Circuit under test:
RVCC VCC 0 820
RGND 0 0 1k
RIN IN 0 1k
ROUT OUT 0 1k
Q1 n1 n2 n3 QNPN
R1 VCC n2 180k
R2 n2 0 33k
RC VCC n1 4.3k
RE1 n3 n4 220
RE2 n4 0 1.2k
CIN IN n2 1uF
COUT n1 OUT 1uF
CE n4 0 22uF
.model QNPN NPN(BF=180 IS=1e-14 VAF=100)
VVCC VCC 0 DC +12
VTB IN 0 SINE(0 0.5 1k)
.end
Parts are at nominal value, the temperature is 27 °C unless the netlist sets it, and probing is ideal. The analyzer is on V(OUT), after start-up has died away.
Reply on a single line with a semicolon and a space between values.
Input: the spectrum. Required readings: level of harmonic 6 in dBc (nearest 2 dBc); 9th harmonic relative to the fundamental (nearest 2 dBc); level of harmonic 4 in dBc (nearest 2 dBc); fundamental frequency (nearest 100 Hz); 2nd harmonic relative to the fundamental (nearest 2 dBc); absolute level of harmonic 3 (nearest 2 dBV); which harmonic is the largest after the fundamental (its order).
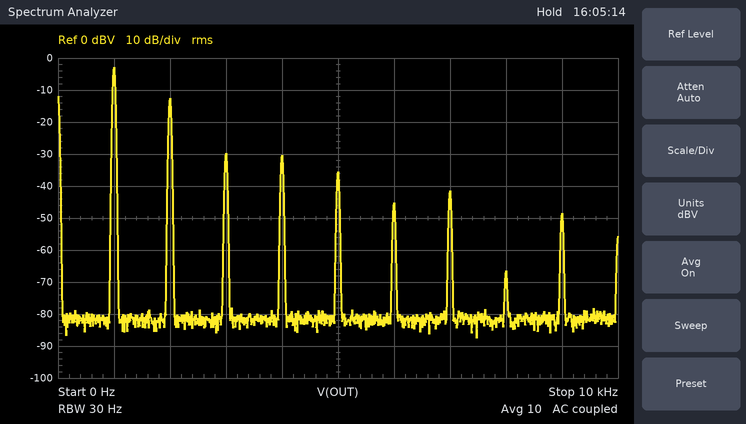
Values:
-42 dBc; -46 dBc; -28 dBc; 1.0 kHz; -10 dBc; -30 dBV; 2
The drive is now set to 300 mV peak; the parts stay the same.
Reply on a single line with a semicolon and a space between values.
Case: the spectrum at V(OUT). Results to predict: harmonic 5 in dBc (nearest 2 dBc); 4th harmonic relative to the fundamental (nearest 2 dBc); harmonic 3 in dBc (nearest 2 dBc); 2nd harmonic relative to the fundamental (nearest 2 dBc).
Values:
-52 dBc; -38 dBc; -26 dBc; -16 dBc
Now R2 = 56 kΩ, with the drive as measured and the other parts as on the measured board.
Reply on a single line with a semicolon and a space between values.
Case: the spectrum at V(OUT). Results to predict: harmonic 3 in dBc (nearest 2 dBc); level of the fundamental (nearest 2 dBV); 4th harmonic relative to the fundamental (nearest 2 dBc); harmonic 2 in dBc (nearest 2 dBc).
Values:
-24 dBc; 0 dBV; -36 dBc; -16 dBc
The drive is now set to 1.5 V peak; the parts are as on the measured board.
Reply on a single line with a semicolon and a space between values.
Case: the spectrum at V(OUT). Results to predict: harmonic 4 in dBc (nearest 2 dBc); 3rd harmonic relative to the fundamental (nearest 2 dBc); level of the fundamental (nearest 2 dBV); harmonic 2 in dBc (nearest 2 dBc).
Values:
-26 dBc; -16 dBc; 2 dBV; -4 dBc
